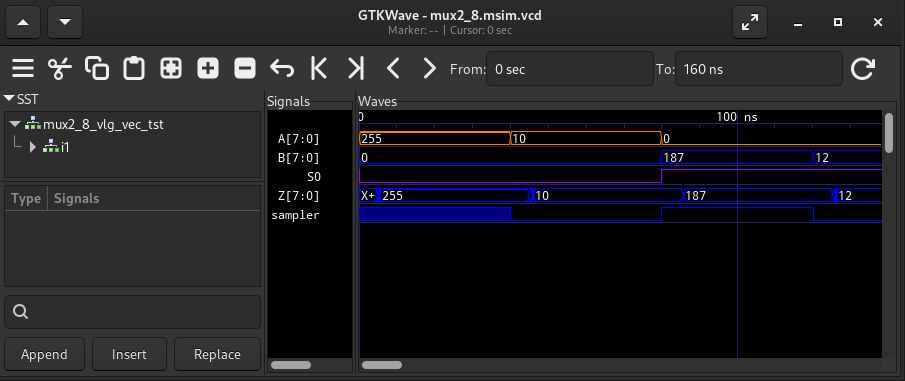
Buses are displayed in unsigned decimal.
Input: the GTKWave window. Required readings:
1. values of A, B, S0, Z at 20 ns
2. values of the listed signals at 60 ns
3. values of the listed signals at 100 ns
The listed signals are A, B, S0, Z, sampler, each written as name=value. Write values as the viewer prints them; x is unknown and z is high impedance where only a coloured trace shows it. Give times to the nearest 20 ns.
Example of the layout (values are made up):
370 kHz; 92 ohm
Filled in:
A=255, B=0, S0=0, Z=255; A=10, B=0, S0=0, Z=10, sampler=0; A=0, B=187, S0=1, Z=187, sampler=1
